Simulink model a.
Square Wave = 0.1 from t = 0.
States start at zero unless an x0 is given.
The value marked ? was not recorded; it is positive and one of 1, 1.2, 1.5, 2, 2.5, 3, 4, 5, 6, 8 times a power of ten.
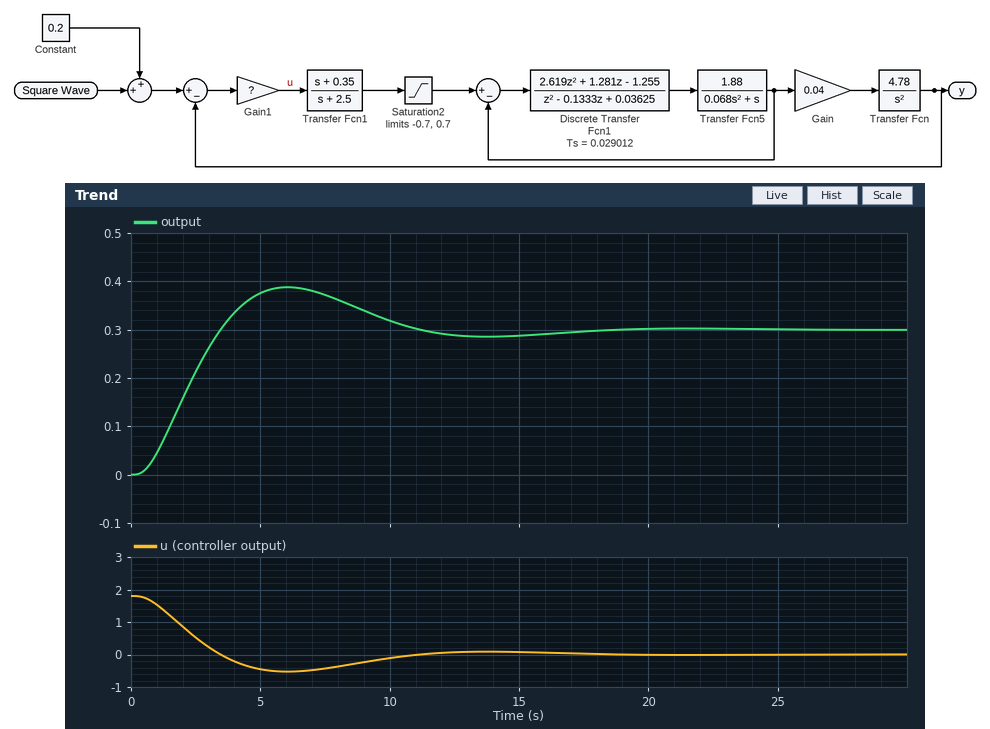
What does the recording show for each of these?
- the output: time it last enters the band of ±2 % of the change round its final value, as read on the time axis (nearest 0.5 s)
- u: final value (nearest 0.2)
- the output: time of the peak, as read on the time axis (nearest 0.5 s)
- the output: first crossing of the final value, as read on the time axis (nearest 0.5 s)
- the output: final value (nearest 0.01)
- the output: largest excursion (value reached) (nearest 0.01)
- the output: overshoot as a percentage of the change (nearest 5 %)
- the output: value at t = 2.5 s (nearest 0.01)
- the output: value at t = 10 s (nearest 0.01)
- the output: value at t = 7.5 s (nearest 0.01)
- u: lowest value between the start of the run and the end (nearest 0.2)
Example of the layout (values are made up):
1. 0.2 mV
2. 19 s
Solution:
1. 17.0 s
2. 0.0
3. 6.0 s
4. 3.5 s
5. 0.30
6. 0.39
7. 30 %
8. 0.21
9. 0.32
10. 0.37
11. -0.6
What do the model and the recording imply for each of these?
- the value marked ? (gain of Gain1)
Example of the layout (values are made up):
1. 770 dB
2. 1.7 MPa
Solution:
1. 6
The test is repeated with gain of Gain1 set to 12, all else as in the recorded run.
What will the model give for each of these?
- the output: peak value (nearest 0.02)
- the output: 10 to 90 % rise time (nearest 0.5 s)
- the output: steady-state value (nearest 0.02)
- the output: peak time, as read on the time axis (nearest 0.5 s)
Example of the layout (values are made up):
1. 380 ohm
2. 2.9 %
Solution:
1. 0.32
2. 2.0 s
3. 0.30
4. 4.5 s
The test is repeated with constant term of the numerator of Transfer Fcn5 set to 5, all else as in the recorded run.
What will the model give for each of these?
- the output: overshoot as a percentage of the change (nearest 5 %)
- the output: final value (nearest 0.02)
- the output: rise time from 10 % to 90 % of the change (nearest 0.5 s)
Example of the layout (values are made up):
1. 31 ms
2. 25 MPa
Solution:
1. 25 %
2. 0.30
3. 2.5 s
